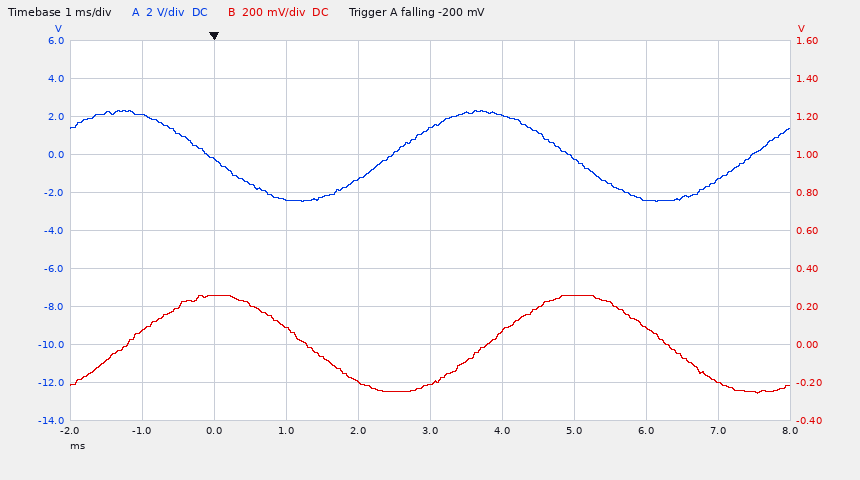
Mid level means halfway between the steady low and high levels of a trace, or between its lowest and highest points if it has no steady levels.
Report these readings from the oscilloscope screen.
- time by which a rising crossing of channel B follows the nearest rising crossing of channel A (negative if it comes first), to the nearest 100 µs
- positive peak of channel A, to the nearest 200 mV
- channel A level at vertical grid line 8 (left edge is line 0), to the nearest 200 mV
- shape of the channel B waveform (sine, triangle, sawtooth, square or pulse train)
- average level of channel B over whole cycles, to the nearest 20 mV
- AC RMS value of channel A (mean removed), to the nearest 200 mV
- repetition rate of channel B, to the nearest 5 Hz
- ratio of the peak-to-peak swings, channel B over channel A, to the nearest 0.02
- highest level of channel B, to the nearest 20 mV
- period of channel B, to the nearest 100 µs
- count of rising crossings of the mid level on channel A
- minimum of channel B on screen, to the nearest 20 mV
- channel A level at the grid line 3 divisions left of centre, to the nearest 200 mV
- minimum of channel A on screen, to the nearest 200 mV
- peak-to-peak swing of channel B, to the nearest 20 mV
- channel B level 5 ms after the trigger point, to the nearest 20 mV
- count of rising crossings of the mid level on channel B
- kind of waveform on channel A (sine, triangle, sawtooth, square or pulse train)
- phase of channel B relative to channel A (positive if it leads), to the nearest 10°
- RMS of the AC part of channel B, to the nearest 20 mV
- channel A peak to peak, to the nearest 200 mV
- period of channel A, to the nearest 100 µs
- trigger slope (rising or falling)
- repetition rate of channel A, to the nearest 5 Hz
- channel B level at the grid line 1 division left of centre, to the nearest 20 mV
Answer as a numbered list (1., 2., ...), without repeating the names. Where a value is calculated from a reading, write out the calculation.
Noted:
1. +1.4 ms
2. 2.4 V
3. -2.4 V
4. sine
5. (260 mV + (-260 mV)) / 2 ≈ 0 mV
6. 4.8 V / (2√2) ≈ 1.70 V, so 1.6 V to the nearest 200 mV
7. 1 / 5.0 ms ≈ 200 Hz
8. 520 mV / 4.8 V ≈ 0.108, so 0.10 to the nearest 0.02
9. 260 mV
10. 5.0 ms
11. 2
12. -260 mV
13. -200 mV
14. -2.4 V
15. 260 mV − (-260 mV) = 520 mV
16. 260 mV
17. 2
18. sine
19. −360° × (+1.4 ms) / 5.0 ms ≈ -101°, so -100° to the nearest 10°
20. 520 mV / (2√2) ≈ 184 mV, so 180 mV to the nearest 20 mV
21. 2.4 V − (-2.4 V) = 4.8 V
22. 5.0 ms
23. falling
24. 1 / 5.0 ms ≈ 200 Hz
25. -200 mV
